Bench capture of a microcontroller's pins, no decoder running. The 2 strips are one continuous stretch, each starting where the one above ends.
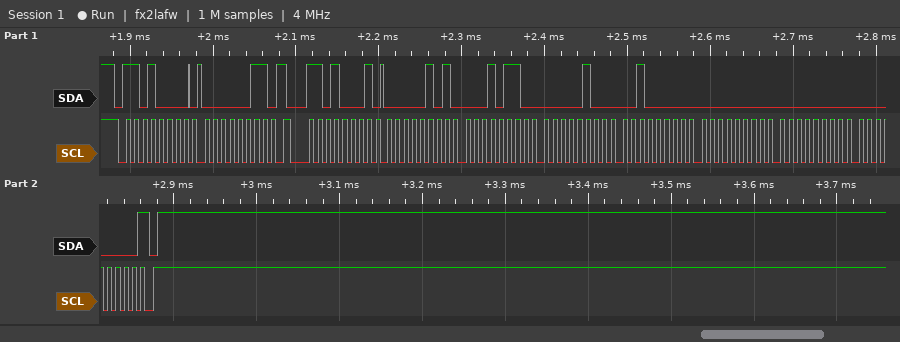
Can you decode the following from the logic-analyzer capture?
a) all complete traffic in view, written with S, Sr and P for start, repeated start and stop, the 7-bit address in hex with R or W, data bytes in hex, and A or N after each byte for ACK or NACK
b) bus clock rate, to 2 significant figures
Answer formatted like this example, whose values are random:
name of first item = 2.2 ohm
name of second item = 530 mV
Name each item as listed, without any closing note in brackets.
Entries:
all complete traffic in view, written with S, Sr and P for start, repeated start and stop, the 7-bit address in hex with R or W, data bytes in hex, and A or N after each byte for ACK or NACK = S 68W A 03 A Sr 68R A 05 A 16 A 04 A 20 A 00 A 00 A 00 N P
bus clock rate, to 2 significant figures = 100 kHz
